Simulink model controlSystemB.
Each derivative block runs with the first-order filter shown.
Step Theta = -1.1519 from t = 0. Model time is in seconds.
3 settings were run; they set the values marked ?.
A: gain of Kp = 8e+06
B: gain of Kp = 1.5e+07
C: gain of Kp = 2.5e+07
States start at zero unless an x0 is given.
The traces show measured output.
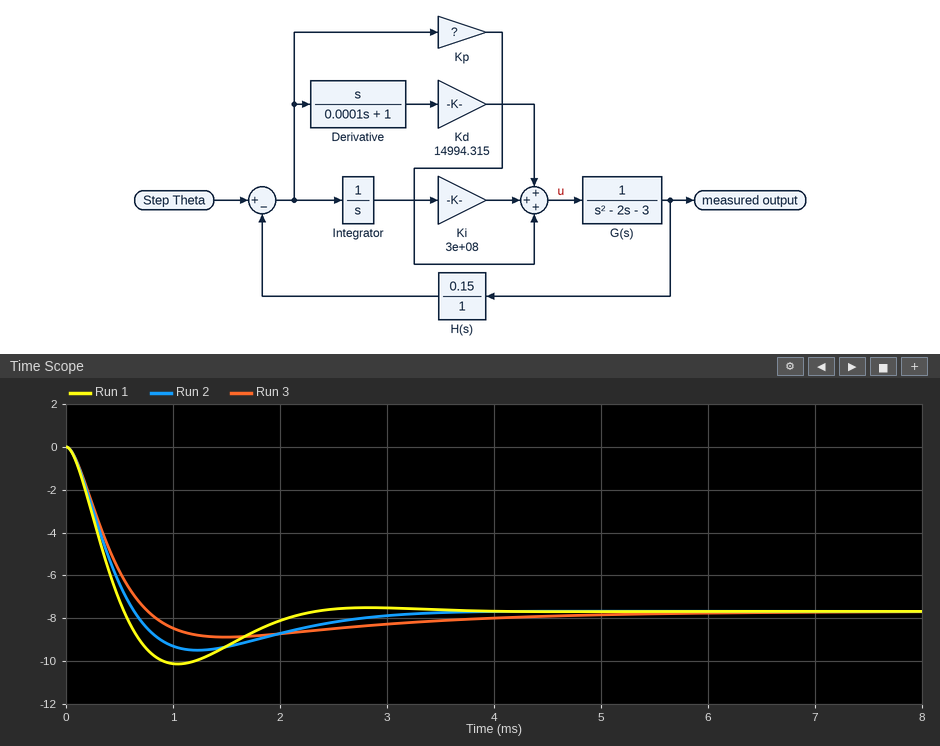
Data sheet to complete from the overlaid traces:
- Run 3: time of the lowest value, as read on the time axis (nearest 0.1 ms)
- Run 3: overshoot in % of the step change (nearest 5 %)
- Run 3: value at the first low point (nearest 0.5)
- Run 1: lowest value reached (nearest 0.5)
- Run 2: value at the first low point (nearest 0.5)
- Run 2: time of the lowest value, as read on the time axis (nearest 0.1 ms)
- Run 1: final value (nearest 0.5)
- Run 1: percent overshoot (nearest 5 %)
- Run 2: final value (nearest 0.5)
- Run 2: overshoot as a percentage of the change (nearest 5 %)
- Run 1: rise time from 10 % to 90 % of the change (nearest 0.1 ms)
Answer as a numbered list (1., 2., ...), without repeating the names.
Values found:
1. 1.5 ms
2. 15 %
3. -9.0
4. -10.0
5. -9.5
6. 1.2 ms
7. -7.5
8. 30 %
9. -7.5
10. 25 %
11. 0.4 ms
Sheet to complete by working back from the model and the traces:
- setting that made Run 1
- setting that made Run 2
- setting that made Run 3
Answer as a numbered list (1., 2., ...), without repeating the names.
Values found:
1. C
2. B
3. A
